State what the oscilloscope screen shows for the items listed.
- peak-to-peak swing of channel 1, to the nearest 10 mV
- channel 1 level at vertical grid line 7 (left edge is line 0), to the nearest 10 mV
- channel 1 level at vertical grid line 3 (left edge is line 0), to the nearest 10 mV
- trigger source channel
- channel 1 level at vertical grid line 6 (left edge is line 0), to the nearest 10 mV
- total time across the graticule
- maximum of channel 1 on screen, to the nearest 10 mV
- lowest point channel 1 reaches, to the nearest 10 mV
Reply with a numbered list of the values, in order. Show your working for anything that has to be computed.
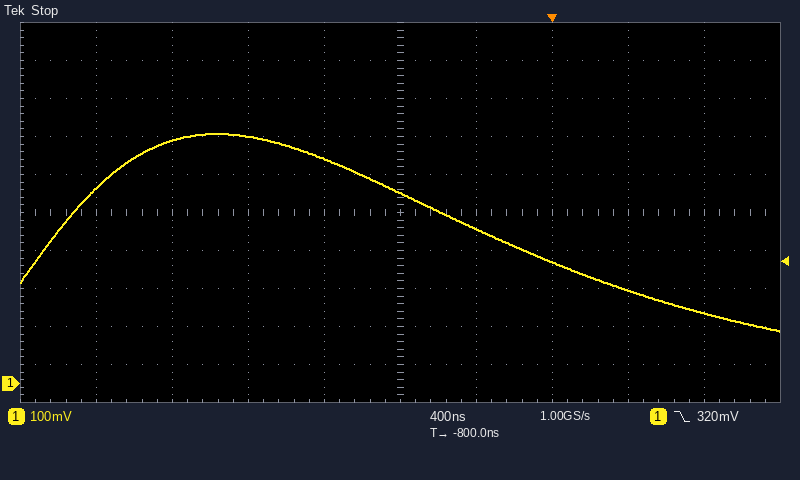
1. 660 mV − (140 mV) = 520 mV
2. 320 mV
3. 650 mV
4. channel 1
5. 410 mV
6. 4 µs
7. 660 mV
8. 140 mV
